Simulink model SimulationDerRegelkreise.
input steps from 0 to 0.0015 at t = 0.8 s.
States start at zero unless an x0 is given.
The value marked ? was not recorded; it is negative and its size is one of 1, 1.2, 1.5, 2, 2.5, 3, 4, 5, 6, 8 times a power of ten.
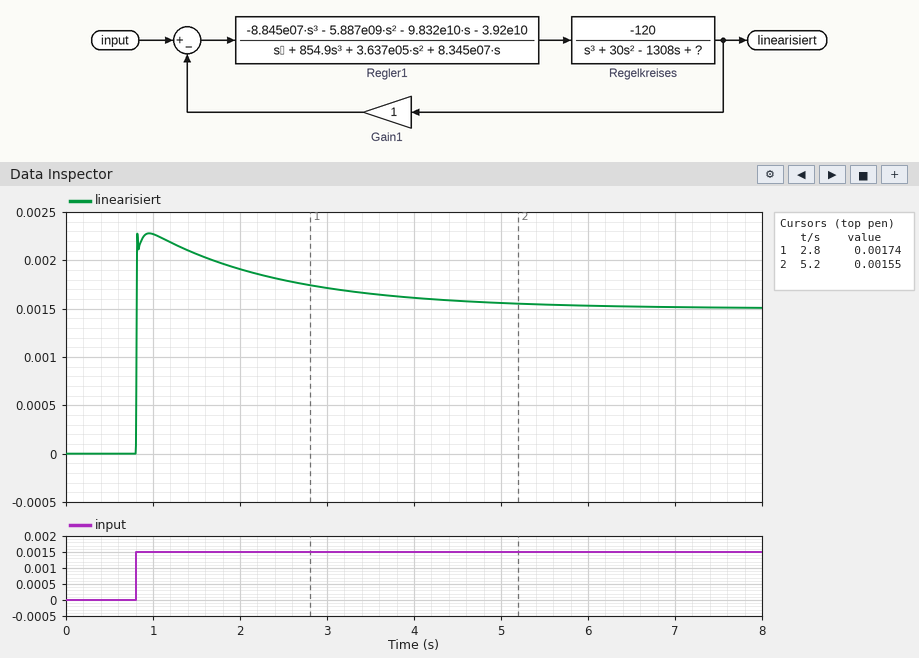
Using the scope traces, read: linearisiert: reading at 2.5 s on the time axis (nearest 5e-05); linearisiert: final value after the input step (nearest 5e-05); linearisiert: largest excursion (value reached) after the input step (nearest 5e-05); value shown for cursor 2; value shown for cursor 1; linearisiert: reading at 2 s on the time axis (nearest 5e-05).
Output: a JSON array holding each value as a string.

["0.00180", "0.00150", "0.00230", "0.00155", "0.00174", "0.00190"]
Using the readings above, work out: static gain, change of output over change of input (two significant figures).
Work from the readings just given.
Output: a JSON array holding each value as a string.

["1.0"]
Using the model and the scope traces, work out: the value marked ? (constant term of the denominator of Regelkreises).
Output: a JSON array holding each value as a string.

["-50000"]
